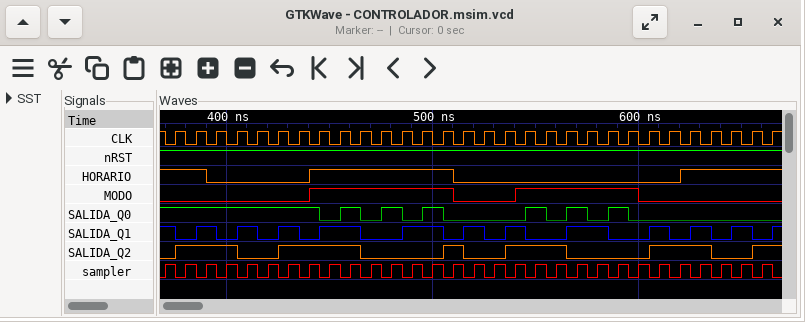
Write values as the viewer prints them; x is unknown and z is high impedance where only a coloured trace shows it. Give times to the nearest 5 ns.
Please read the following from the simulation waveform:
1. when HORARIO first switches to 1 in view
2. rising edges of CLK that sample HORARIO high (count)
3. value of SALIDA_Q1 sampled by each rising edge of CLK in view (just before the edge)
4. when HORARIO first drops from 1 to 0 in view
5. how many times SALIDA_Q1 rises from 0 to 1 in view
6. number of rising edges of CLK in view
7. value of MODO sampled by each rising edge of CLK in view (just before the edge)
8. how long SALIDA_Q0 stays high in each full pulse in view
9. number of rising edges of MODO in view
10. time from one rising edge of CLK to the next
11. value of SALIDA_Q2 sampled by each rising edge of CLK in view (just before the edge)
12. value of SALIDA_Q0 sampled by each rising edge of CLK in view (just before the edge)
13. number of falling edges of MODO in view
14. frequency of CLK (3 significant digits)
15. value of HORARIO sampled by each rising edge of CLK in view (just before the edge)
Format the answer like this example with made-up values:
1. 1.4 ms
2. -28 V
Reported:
1. 440 ns
2. 14
3. 1 0 1 0 1 0 1 0 1 1 0 0 1 1 0 1 0 1 0 0 1 1 0 0 1 0 1 0 1 0
4. 390 ns
5. 12
6. 30
7. 0 0 0 0 0 0 0 1 1 1 1 1 1 1 0 0 0 1 1 1 1 1 1 0 0 0 0 0 0 0
8. 10 ns, 10 ns, 10 ns, 10 ns, 10 ns, 10 ns
9. 2
10. 10 ns
11. 0 1 1 1 0 0 1 1 1 1 0 0 0 0 1 0 0 1 1 1 0 0 0 0 1 1 1 0 0 1
12. 1 1 1 1 1 1 1 1 0 1 0 1 0 1 0 0 0 0 1 0 1 0 1 0 0 0 0 0 0 0
13. 2
14. 100 MHz
15. 1 1 0 0 0 0 0 1 1 1 1 1 1 1 0 0 0 0 0 0 0 0 0 0 0 1 1 1 1 1
